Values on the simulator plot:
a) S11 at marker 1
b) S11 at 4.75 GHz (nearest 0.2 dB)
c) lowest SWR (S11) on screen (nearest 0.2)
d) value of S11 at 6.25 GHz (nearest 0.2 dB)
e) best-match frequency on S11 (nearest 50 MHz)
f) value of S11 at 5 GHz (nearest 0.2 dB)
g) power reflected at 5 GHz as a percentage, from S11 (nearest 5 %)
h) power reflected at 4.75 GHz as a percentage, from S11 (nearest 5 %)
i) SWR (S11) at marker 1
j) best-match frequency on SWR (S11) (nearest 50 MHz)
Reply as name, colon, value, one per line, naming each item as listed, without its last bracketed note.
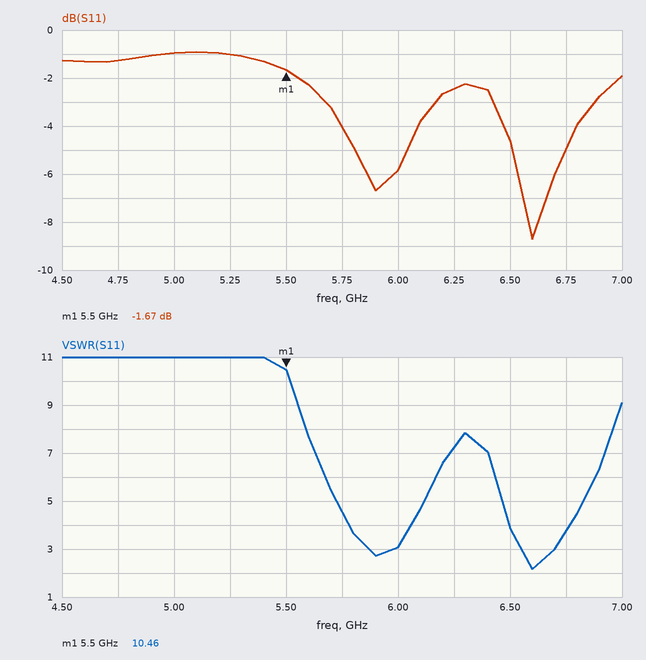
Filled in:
S11 at marker 1: -1.67 dB
S11 at 4.75 GHz: -1.2 dB
lowest SWR (S11) on screen: 2.2
value of S11 at 6.25 GHz: -2.4 dB
best-match frequency on S11: 6.60 GHz
value of S11 at 5 GHz: -1.0 dB
power reflected at 5 GHz as a percentage, from S11: 80 %
power reflected at 4.75 GHz as a percentage, from S11: 75 %
SWR (S11) at marker 1: 10.46
best-match frequency on SWR (S11): 6.60 GHz
